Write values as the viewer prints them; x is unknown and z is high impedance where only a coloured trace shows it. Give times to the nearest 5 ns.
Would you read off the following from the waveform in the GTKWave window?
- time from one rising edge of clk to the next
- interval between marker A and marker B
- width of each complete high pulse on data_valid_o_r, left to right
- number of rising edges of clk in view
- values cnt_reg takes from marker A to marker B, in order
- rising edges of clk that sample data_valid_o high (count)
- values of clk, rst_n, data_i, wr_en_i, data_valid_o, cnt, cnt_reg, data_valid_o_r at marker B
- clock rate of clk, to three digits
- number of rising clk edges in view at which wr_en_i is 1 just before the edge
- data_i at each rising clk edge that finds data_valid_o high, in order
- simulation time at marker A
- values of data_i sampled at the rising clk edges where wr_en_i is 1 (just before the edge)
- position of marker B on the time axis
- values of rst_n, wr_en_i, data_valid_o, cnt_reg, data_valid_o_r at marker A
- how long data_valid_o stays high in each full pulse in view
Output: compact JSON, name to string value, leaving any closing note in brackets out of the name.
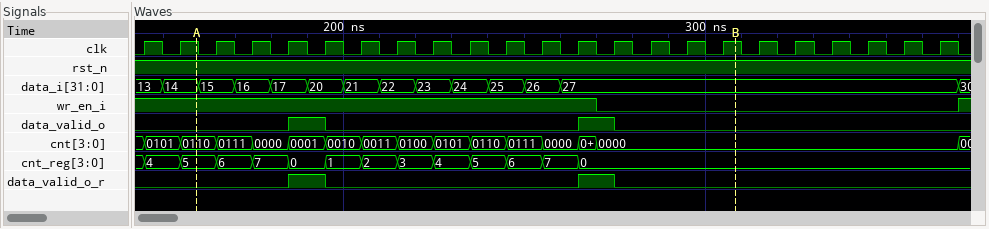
{"time from one rising edge of clk to the next": "10 ns", "interval between marker A and marker B": "150 ns", "width of each complete high pulse on data_valid_o_r, left to right": "10 ns, 10 ns", "number of rising edges of clk in view": "23", "values cnt_reg takes from marker A to marker B, in order": "5, 6, 7, 0, 1, 2, 3, 4, 5, 6, 7, 0", "rising edges of clk that sample data_valid_o high": "2", "values of clk, rst_n, data_i, wr_en_i, data_valid_o, cnt, cnt_reg, data_valid_o_r at marker B": "clk=1, rst_n=1, data_i=27, wr_en_i=0, data_valid_o=0, cnt=0000, cnt_reg=0, data_valid_o_r=0", "clock rate of clk, to three digits": "100 MHz", "number of rising clk edges in view at which wr_en_i is 1 just before the edge": "13", "data_i at each rising clk edge that finds data_valid_o high, in order": "20, 27", "simulation time at marker A": "160 ns", "values of data_i sampled at the rising clk edges where wr_en_i is 1": "13, 14, 15, 16, 17, 20, 21, 22, 23, 24, 25, 26, 27", "position of marker B on the time axis": "310 ns", "values of rst_n, wr_en_i, data_valid_o, cnt_reg, data_valid_o_r at marker A": "rst_n=1, wr_en_i=1, data_valid_o=0, cnt_reg=5, data_valid_o_r=0", "how long data_valid_o stays high in each full pulse in view": "10 ns, 10 ns"}
